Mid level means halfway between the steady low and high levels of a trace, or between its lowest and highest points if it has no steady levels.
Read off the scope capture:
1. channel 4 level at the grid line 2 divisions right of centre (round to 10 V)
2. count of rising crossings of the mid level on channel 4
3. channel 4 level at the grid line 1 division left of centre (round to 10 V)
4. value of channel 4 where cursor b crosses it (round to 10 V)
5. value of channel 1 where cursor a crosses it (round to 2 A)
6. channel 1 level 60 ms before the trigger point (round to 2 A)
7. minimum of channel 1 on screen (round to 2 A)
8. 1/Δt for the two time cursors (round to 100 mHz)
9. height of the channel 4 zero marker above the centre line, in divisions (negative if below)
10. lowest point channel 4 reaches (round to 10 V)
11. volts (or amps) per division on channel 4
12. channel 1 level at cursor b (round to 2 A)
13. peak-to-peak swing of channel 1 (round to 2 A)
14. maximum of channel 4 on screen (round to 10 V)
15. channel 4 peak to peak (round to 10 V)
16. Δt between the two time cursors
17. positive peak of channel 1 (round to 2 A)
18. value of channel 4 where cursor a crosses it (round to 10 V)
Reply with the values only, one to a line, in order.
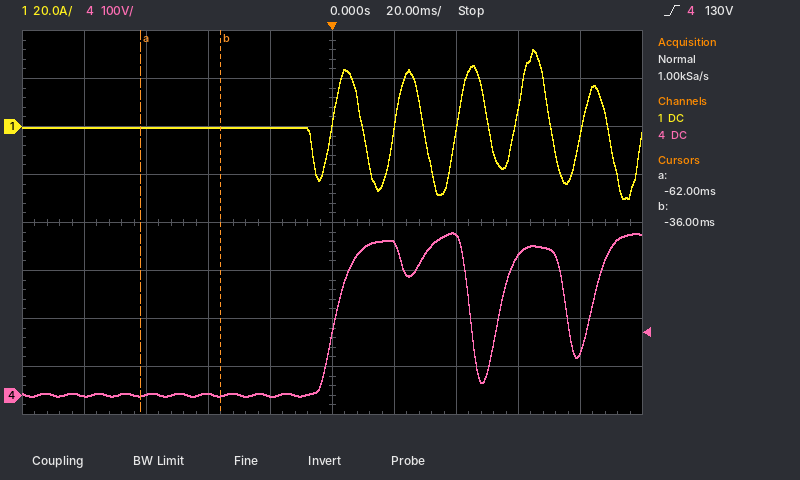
330 V
3
0 V
0 V
0 A
0 A
-30 A
38.5 Hz
-3.6 div
0 V
100 V
0 A
62 A
340 V
340 V
26 ms
32 A
0 V
